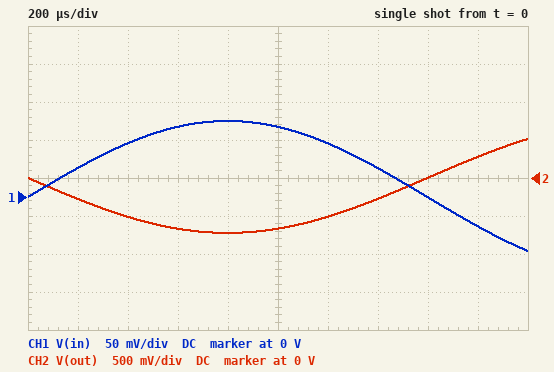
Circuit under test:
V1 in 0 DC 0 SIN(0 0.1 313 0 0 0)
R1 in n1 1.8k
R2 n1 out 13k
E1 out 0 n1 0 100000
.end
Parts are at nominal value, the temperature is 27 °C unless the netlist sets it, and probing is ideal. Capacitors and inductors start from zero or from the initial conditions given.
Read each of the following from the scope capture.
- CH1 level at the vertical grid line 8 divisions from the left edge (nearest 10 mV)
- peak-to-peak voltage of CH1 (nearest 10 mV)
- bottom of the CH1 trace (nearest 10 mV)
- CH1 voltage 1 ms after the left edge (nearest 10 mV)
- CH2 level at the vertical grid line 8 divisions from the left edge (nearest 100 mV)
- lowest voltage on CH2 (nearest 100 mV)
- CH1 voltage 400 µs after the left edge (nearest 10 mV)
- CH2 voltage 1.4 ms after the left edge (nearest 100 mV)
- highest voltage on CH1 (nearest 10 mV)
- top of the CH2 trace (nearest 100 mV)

0 V
170 mV
-70 mV
90 mV
0 V
-700 mV
70 mV
-300 mV
100 mV
500 mV
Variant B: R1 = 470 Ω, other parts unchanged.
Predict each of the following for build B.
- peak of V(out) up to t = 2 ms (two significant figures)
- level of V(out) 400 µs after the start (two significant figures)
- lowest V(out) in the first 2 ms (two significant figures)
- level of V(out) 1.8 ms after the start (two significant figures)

2.0 V
-2.0 V
-2.8 V
1.1 V
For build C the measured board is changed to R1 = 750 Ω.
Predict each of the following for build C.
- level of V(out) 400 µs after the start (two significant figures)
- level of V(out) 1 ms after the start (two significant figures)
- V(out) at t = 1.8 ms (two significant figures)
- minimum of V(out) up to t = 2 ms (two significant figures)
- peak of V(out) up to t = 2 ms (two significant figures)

-1.2 V
-1.6 V
670 mV
-1.7 V
1.2 V
